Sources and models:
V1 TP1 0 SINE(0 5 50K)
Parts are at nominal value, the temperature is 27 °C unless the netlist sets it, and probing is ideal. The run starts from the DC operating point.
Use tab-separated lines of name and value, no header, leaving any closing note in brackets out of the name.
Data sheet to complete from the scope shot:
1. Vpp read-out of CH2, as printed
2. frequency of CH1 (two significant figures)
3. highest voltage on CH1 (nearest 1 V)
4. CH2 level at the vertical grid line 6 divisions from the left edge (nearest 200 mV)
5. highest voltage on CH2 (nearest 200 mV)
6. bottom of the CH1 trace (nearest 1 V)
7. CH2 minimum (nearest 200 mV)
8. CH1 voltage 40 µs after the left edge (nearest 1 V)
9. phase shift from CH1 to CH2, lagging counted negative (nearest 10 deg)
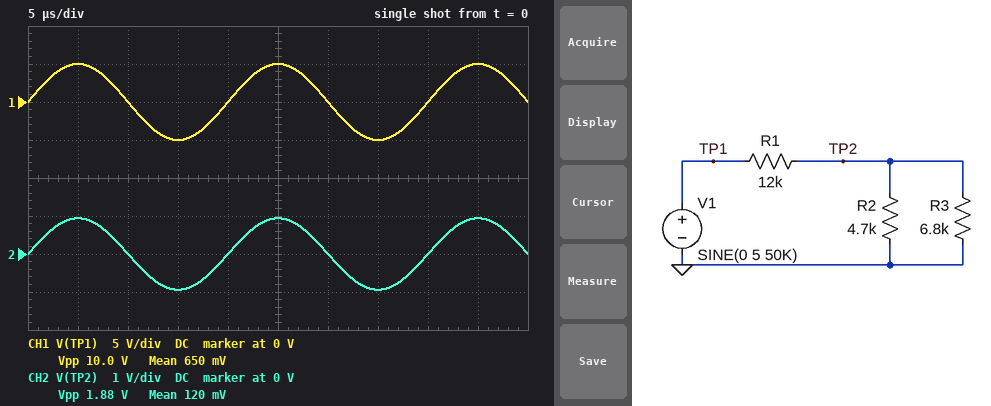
Vpp read-out of CH2, as printed	1.88 V
frequency of CH1	50 kHz
highest voltage on CH1	5 V
CH2 level at the vertical grid line 6 divisions from the left edge	0 V
highest voltage on CH2	1.0 V
bottom of the CH1 trace	-5 V
CH2 minimum	-1.0 V
CH1 voltage 40 µs after the left edge	0 V
phase shift from CH1 to CH2, lagging counted negative	0 deg
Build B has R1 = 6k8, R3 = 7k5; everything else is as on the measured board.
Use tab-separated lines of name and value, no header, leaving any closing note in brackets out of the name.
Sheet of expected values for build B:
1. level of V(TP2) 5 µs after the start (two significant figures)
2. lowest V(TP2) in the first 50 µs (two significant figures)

level of V(TP2) 5 µs after the start	1.5 V
lowest V(TP2) in the first 50 µs	-1.5 V
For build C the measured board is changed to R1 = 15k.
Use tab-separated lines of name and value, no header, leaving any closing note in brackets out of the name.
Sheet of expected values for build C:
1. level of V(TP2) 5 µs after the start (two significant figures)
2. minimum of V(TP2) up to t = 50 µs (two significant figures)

level of V(TP2) 5 µs after the start	780 mV
minimum of V(TP2) up to t = 50 µs	-780 mV
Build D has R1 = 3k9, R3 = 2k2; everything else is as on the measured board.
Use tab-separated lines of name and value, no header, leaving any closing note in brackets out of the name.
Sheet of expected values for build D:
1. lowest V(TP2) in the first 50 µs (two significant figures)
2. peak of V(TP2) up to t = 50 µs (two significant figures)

lowest V(TP2) in the first 50 µs	-1.4 V
peak of V(TP2) up to t = 50 µs	1.4 V
